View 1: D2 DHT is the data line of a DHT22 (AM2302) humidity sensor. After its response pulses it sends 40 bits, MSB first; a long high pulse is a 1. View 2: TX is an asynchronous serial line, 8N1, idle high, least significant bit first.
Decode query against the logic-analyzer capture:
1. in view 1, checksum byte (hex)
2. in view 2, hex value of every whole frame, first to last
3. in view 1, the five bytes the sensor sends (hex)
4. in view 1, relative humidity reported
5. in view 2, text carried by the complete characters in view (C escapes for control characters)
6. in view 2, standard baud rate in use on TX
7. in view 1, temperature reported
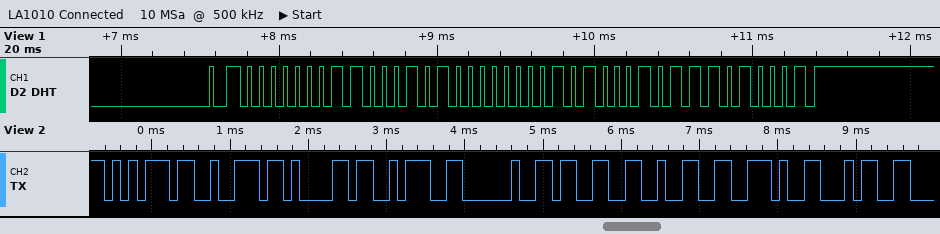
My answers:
0xD1
75 72 61 3A 20 33 32 2E 34
01 8A 01 45 D1
39.4 %
"ura: 32.4"
9600 baud
32.5 °C
